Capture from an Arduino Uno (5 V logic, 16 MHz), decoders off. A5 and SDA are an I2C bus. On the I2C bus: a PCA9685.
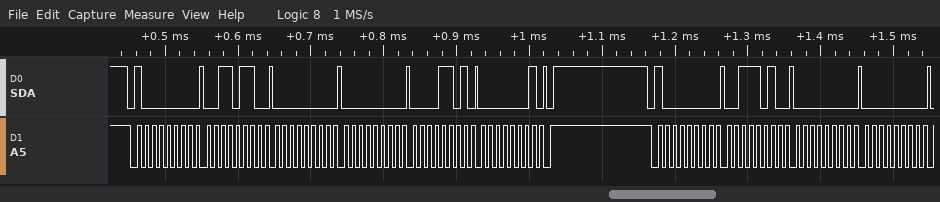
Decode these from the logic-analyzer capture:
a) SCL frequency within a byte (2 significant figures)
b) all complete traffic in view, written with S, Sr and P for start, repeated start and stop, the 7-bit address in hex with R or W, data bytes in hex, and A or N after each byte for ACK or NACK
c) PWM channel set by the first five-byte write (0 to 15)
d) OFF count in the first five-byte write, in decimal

100 kHz
S 40W A 36 A 00 A 00 A 0D A 01 A P S 40W A 3A A 00 A 00 A
12
269
